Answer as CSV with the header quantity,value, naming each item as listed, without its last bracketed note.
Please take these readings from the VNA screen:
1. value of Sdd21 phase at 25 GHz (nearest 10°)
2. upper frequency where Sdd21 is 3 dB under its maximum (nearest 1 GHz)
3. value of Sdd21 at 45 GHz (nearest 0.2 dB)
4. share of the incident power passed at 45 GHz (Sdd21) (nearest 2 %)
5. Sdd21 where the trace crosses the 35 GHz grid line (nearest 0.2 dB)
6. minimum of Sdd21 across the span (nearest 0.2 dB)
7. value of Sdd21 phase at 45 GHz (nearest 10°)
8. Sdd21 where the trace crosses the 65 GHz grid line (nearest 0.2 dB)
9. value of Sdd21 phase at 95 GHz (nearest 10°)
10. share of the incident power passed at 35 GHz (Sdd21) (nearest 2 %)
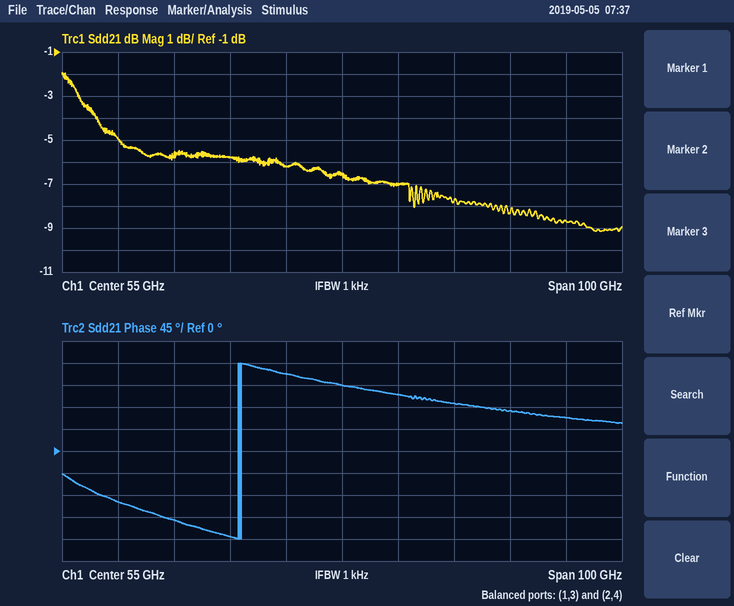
quantity,value
value of Sdd21 phase at 25 GHz,-140°
upper frequency where Sdd21 is 3 dB under its maximum,15 GHz
value of Sdd21 at 45 GHz,-6.2 dB
share of the incident power passed at 45 GHz (Sdd21),24 %
Sdd21 where the trace crosses the 35 GHz grid line,-5.8 dB
minimum of Sdd21 across the span,-9.2 dB
value of Sdd21 phase at 45 GHz,160°
Sdd21 where the trace crosses the 65 GHz grid line,-7.0 dB
value of Sdd21 phase at 95 GHz,70°
share of the incident power passed at 35 GHz (Sdd21),26 %
